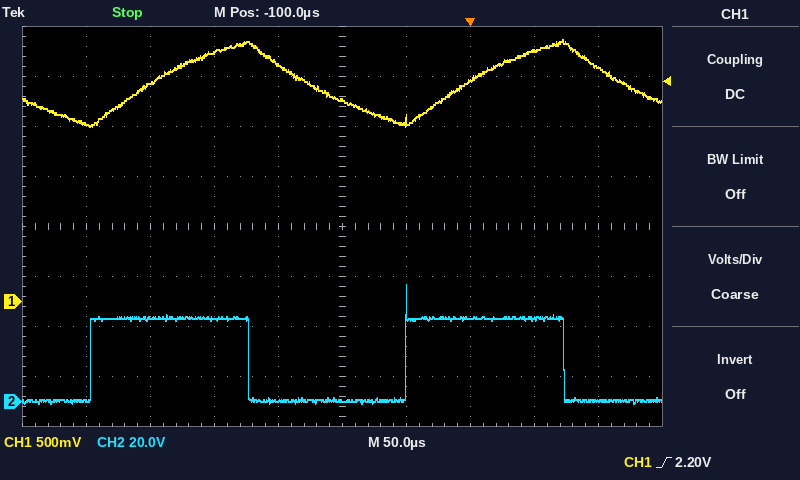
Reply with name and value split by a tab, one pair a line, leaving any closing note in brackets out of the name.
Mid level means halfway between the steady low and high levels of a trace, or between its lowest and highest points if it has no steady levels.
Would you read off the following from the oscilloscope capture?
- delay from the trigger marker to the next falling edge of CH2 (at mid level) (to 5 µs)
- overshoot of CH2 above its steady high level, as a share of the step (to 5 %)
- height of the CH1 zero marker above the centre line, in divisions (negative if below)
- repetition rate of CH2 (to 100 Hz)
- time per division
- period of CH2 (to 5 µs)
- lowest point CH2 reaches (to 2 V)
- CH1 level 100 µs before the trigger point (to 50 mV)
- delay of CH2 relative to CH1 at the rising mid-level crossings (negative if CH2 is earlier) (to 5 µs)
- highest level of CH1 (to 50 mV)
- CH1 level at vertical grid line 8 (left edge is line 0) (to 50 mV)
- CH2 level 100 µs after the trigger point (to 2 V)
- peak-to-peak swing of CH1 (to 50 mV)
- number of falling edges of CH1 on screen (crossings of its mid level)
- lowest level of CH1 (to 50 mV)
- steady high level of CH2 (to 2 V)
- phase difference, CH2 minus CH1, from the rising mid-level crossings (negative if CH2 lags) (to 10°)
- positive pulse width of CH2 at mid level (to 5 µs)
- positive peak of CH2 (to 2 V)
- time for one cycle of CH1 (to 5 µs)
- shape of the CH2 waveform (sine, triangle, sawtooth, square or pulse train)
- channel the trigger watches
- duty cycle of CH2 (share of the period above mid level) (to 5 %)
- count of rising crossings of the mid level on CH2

delay from the trigger marker to the next falling edge of CH2 (at mid level)	75 µs
overshoot of CH2 above its steady high level, as a share of the step	40 %
height of the CH1 zero marker above the centre line, in divisions	-1.5 div
repetition rate of CH2	4.1 kHz
time per division	50 µs
period of CH2	245 µs
lowest point CH2 reaches	0 V
CH1 level 100 µs before the trigger point	2.00 V
delay of CH2 relative to CH1 at the rising mid-level crossings (negative if CH2 is earlier)	-50 µs
highest level of CH1	2.60 V
CH1 level at vertical grid line 8 (left edge is line 0)	2.50 V
CH2 level 100 µs after the trigger point	0 V
peak-to-peak swing of CH1	850 mV
number of falling edges of CH1 on screen	2
lowest level of CH1	1.75 V
steady high level of CH2	34 V
phase difference, CH2 minus CH1, from the rising mid-level crossings (negative if CH2 lags)	+70°
positive pulse width of CH2 at mid level	125 µs
positive peak of CH2	46 V
time for one cycle of CH1	245 µs
shape of the CH2 waveform	square
channel the trigger watches	CH1
duty cycle of CH2 (share of the period above mid level)	50 %
count of rising crossings of the mid level on CH2	2
